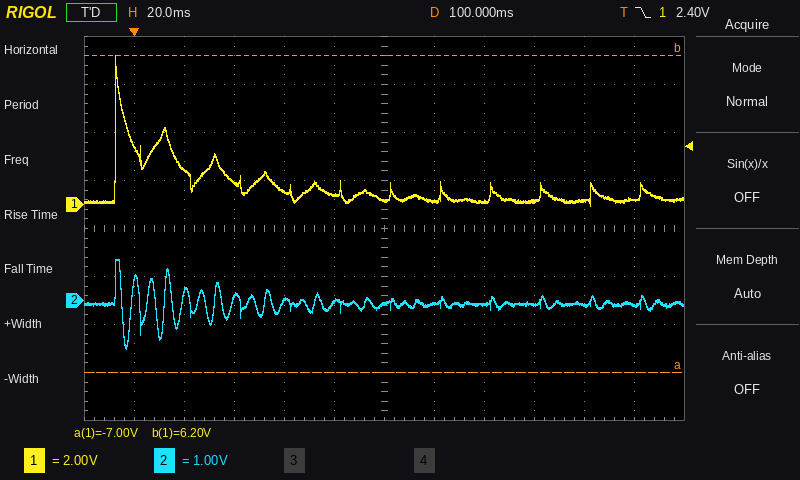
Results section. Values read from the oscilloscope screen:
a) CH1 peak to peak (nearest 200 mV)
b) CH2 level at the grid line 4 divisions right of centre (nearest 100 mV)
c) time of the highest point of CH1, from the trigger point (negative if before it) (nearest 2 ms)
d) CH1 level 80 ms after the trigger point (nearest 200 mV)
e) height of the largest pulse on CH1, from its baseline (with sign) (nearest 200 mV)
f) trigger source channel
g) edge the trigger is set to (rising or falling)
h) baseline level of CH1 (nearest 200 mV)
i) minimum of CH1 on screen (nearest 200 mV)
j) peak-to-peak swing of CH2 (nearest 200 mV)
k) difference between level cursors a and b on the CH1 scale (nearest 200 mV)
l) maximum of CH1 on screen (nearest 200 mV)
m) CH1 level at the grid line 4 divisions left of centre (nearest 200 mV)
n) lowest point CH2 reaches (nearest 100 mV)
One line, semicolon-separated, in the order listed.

6.2 V; -100 mV; -8 ms; 400 mV; +6.0 V; CH1; falling; 200 mV; 0.0 V; 1.8 V; 13.2 V; 6.2 V; 1.4 V; -1.0 V
